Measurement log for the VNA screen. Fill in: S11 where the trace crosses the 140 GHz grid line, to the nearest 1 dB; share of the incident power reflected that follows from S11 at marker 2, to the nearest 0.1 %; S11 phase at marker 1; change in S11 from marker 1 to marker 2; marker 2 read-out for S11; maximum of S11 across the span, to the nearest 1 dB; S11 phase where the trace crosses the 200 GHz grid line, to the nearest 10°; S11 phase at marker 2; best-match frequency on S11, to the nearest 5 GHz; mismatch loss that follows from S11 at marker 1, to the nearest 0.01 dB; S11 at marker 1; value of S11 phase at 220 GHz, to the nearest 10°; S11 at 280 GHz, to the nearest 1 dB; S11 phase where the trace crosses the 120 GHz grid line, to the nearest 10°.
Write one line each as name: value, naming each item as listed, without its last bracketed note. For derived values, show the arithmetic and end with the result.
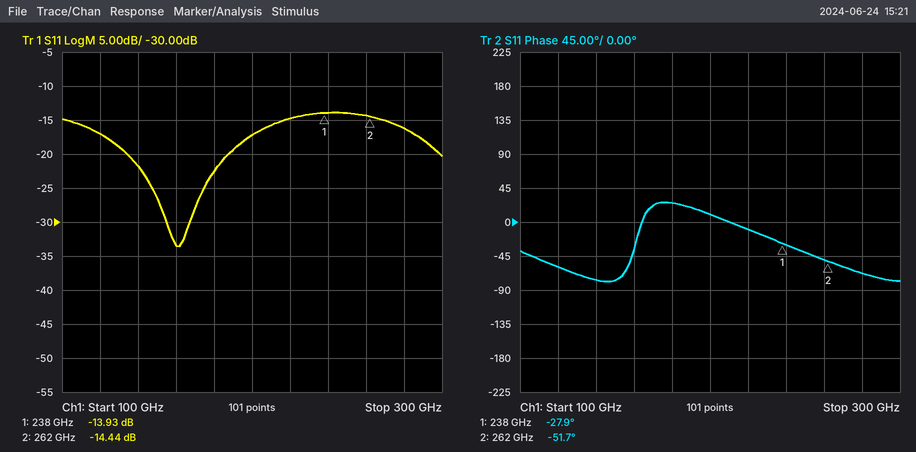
S11 where the trace crosses the 140 GHz grid line, to the nearest 1 dB: -22 dB
share of the incident power reflected that follows from S11 at marker 2, to the nearest 0.1 %: 10^(-14.44/10) ≈ 3.6 %
S11 phase at marker 1: -27.9°
change in S11 from marker 1 to marker 2: -14.44 − (-13.93) = -0.51 dB
marker 2 read-out for S11: -14.44 dB
maximum of S11 across the span, to the nearest 1 dB: -14 dB
S11 phase where the trace crosses the 200 GHz grid line, to the nearest 10°: 10°
S11 phase at marker 2: -51.7°
best-match frequency on S11, to the nearest 5 GHz: 160 GHz
mismatch loss that follows from S11 at marker 1, to the nearest 0.01 dB: −10 log10(1 − 10^(-13.93/10)) ≈ 0.18 dB
S11 at marker 1: -13.93 dB
value of S11 phase at 220 GHz, to the nearest 10°: -10°
S11 at 280 GHz, to the nearest 1 dB: -16 dB
S11 phase where the trace crosses the 120 GHz grid line, to the nearest 10°: -60°
